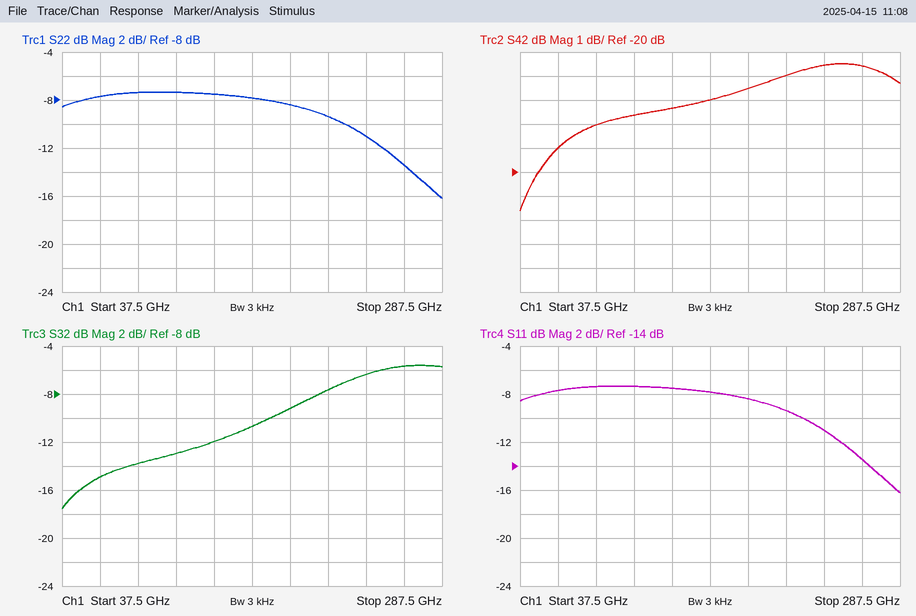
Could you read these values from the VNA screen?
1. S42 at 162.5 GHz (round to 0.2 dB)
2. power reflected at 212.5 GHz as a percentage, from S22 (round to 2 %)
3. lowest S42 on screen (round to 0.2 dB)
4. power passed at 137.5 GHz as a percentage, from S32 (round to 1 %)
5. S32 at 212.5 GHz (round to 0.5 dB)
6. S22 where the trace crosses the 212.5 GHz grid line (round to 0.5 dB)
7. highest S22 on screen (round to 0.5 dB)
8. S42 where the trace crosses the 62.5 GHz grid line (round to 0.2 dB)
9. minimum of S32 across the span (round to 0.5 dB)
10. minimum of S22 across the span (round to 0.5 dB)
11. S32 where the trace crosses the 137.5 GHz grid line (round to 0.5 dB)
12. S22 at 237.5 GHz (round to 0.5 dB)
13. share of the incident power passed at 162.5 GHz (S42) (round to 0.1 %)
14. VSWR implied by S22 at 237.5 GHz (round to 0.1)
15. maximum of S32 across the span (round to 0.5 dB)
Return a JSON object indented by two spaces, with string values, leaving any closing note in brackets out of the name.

{
  "S42 at 162.5 GHz": "-17.0 dB",
  "power reflected at 212.5 GHz as a percentage, from S22": "12 %",
  "lowest S42 on screen": "-21.6 dB",
  "power passed at 137.5 GHz as a percentage, from S32": "6 %",
  "S32 at 212.5 GHz": "-7.5 dB",
  "S22 where the trace crosses the 212.5 GHz grid line": "-9.5 dB",
  "highest S22 on screen": "-7.5 dB",
  "S42 where the trace crosses the 62.5 GHz grid line": "-19.0 dB",
  "minimum of S32 across the span": "-17.5 dB",
  "minimum of S22 across the span": "-16.0 dB",
  "S32 where the trace crosses the 137.5 GHz grid line": "-12.0 dB",
  "S22 at 237.5 GHz": "-11.0 dB",
  "share of the incident power passed at 162.5 GHz (S42)": "2.0 %",
  "VSWR implied by S22 at 237.5 GHz": "1.8",
  "maximum of S32 across the span": "-5.5 dB"
}
